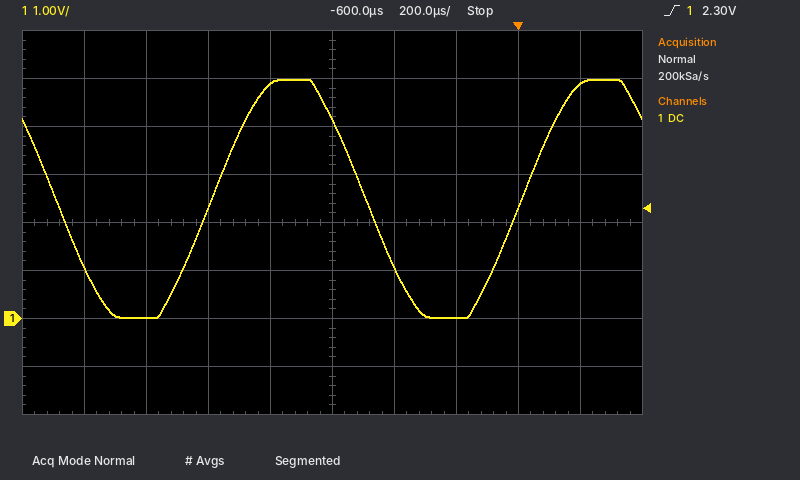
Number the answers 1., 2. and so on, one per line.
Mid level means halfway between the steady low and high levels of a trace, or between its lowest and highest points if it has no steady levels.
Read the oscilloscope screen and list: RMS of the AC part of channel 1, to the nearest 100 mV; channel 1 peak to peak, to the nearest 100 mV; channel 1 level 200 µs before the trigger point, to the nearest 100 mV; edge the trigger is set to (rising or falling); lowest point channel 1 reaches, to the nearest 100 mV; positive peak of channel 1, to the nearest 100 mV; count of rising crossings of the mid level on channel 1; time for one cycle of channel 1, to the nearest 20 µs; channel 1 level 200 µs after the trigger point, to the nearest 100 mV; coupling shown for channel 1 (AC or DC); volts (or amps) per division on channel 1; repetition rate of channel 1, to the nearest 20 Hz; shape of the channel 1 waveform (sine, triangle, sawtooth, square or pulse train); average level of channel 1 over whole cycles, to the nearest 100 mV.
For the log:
1. 1.8 V
2. 5.0 V
3. 0.0 V
4. rising
5. 0.0 V
6. 5.0 V
7. 2
8. 1.00 ms
9. 4.9 V
10. DC
11. 1 V
12. 1.00 kHz
13. sine
14. 2.5 V
